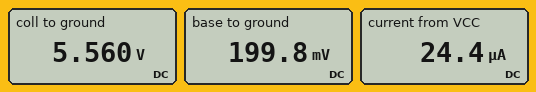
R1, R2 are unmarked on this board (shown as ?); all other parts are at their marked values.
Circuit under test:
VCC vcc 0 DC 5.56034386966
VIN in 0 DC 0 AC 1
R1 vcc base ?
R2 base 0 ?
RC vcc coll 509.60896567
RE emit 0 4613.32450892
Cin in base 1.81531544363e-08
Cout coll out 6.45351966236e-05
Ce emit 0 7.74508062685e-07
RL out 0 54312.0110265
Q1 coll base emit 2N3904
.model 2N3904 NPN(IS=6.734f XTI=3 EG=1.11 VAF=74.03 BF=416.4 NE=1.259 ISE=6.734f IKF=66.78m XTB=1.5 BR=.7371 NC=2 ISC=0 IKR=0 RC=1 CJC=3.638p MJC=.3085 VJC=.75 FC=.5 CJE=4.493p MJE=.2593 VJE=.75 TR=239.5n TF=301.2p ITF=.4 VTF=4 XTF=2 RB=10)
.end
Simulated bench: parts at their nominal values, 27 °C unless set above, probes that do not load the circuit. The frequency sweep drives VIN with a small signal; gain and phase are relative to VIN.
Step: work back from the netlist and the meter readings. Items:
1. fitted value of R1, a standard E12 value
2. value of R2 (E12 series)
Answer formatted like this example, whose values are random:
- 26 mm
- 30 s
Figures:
- 220 kΩ
- 8.2 kΩ
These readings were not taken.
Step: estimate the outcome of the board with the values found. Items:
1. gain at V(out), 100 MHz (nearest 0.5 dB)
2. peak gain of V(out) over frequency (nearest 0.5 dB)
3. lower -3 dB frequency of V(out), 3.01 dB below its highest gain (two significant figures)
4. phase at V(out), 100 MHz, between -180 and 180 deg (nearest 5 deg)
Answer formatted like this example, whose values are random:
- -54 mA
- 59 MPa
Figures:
- -6.0 dB
- -0.5 dB
- 150 MHz
- 55 deg
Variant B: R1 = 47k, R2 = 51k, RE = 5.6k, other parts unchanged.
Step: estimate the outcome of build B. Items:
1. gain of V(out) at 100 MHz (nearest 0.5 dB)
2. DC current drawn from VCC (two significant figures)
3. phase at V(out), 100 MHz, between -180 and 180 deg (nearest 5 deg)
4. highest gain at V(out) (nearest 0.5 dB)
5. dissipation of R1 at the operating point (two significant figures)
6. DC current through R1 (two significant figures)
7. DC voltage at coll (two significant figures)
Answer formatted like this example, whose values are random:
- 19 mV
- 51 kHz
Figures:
- 15.0 dB
- 440 µA
- 130 deg
- 17.5 dB
- 160 µW
- 58 µA
- 5.4 V
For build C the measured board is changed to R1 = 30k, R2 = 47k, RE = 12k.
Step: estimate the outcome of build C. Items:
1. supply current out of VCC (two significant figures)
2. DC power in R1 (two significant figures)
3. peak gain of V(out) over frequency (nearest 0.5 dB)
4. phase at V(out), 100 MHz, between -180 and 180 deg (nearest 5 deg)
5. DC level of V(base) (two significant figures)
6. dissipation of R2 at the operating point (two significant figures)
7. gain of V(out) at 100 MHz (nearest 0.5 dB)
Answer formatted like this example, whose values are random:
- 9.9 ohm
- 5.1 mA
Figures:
- 300 µA
- 160 µW
- 13.0 dB
- 125 deg
- 3.4 V
- 240 µW
- 10.5 dB
